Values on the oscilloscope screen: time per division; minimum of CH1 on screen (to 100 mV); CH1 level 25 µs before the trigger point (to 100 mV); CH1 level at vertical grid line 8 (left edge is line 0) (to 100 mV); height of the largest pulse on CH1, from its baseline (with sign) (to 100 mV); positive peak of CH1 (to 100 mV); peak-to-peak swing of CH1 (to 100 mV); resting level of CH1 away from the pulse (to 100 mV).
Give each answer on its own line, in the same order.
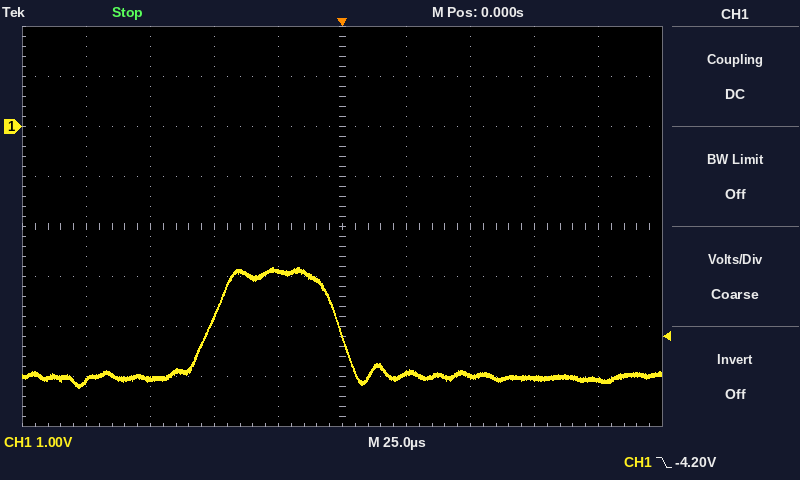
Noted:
25 µs
-5.2 V
-2.9 V
-5.0 V
+2.2 V
-2.8 V
2.4 V
-5.0 V
